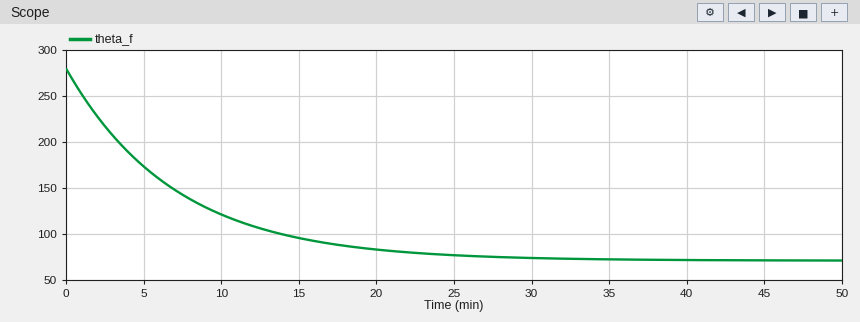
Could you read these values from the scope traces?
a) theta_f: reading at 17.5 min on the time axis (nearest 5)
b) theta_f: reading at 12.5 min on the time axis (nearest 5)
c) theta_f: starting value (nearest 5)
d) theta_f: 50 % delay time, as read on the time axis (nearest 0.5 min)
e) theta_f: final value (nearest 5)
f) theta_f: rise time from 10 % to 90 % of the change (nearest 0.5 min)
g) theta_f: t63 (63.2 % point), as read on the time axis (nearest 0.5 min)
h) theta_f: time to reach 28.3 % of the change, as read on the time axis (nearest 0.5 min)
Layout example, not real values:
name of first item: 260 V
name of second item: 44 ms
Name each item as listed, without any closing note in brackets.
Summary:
theta_f: reading at 17.5 min on the time axis: 90
theta_f: reading at 12.5 min on the time axis: 105
theta_f: starting value: 280
theta_f: 50 % delay time, as read on the time axis: 5.0 min
theta_f: final value: 70
theta_f: rise time from 10 % to 90 % of the change: 15.5 min
theta_f: t63 (63.2 % point), as read on the time axis: 7.0 min
theta_f: time to reach 28.3 % of the change, as read on the time axis: 2.5 min
